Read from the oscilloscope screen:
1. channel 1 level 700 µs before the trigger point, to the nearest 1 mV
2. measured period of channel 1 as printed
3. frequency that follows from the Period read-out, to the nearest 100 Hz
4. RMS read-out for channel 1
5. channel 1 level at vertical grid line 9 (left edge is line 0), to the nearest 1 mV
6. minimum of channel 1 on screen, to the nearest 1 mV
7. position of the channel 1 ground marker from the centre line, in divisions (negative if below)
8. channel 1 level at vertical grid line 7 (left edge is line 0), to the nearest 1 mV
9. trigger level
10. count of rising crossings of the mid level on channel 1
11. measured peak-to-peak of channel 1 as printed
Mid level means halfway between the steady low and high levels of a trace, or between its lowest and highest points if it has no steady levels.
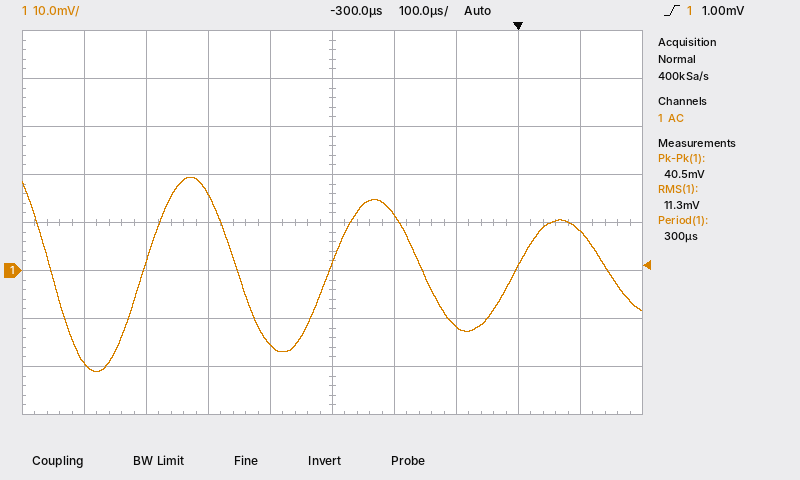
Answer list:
-19 mV
300 µs
3.3 kHz
11.3 mV
8 mV
-21 mV
-1.0 div
-12 mV
1.00 mV
3
40.5 mV
